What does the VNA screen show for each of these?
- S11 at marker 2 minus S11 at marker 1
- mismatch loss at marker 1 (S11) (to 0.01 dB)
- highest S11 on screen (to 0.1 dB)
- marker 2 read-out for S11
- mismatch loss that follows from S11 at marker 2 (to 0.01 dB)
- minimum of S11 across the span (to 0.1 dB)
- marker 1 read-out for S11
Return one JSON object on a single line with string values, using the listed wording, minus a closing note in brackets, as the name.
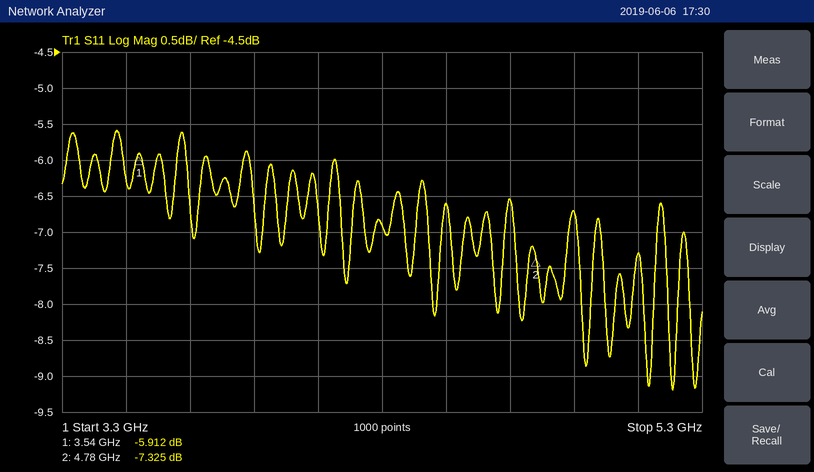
{"S11 at marker 2 minus S11 at marker 1": "-1.413 dB", "mismatch loss at marker 1 (S11)": "1.29 dB", "highest S11 on screen": "-5.6 dB", "marker 2 read-out for S11": "-7.325 dB", "mismatch loss that follows from S11 at marker 2": "0.89 dB", "minimum of S11 across the span": "-9.2 dB", "marker 1 read-out for S11": "-5.912 dB"}
